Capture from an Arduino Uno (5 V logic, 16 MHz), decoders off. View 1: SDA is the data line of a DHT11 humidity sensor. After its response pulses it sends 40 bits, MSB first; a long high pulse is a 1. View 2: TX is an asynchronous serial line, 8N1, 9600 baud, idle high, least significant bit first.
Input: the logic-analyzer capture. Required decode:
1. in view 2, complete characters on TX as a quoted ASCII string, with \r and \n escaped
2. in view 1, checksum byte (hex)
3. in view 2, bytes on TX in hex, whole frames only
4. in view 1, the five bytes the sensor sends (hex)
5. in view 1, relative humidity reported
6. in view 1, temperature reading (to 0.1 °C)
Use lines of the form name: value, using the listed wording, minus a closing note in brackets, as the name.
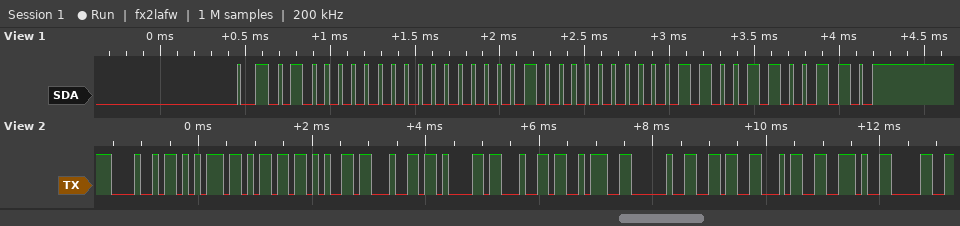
in view 2, complete characters on TX as a quoted ASCII string, with \r and \n escaped: "Humedad: 64.0"
in view 1, checksum byte: 0x66
in view 2, bytes on TX in hex, whole frames only: 48 75 6D 65 64 61 64 3A 20 36 34 2E 30
in view 1, the five bytes the sensor sends: 40 00 20 06 66
in view 1, relative humidity reported: 64 %
in view 1, temperature reading: 32.6 °C
